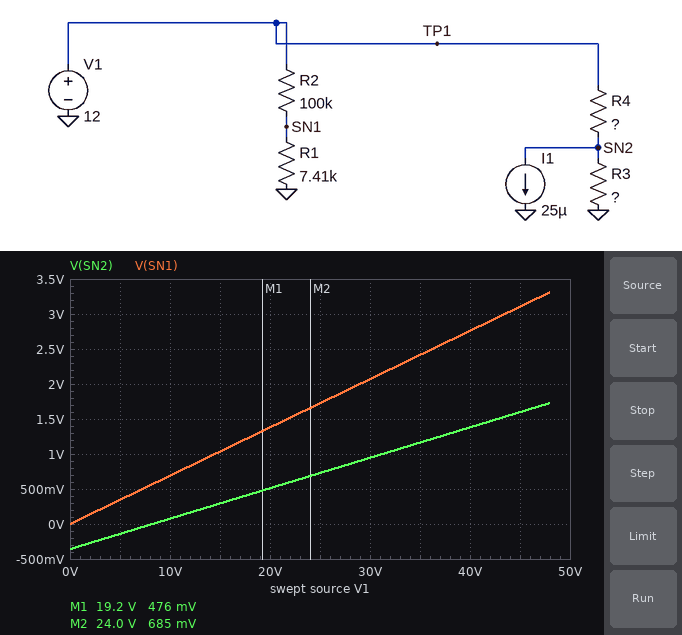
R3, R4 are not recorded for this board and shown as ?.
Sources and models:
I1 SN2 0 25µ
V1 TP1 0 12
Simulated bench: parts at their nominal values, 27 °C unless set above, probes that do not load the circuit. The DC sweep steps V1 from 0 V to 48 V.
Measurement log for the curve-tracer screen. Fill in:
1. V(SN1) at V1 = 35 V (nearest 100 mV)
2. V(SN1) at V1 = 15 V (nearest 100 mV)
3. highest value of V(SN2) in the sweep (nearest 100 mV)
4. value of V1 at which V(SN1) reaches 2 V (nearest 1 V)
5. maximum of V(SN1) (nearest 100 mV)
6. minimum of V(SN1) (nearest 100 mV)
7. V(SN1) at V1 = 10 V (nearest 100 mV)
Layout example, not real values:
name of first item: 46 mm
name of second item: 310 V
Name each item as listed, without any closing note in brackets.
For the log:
V(SN1) at V1 = 35 V: 2.4 V
V(SN1) at V1 = 15 V: 1.0 V
highest value of V(SN2) in the sweep: 1.7 V
value of V1 at which V(SN1) reaches 2 V: 29 V
maximum of V(SN1): 3.3 V
minimum of V(SN1): 0 V
V(SN1) at V1 = 10 V: 700 mV
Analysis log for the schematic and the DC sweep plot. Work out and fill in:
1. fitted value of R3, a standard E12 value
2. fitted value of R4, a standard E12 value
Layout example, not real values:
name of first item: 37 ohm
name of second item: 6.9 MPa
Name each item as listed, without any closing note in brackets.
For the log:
fitted value of R3, a standard E12 value: 15 kΩ
fitted value of R4, a standard E12 value: 330 kΩ
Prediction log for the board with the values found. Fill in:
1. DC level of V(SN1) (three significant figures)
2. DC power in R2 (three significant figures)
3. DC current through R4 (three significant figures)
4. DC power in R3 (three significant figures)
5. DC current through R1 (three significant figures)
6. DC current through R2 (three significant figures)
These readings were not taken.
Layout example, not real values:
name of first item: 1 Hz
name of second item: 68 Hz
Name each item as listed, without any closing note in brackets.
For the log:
DC level of V(SN1): 828 mV
DC power in R2: 1.25 mW
DC current through R4: 35.9 µA
DC power in R3: 1.77 µW
DC current through R1: 112 µA
DC current through R2: 112 µA
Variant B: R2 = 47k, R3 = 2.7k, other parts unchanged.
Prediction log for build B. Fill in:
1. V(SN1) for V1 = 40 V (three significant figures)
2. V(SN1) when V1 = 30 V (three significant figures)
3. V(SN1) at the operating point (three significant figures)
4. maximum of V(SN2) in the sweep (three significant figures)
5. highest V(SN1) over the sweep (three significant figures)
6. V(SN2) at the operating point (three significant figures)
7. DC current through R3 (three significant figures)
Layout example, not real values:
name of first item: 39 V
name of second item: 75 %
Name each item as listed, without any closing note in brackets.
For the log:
V(SN1) for V1 = 40 V: 5.45 V
V(SN1) when V1 = 30 V: 4.09 V
V(SN1) at the operating point: 1.63 V
maximum of V(SN2) in the sweep: 323 mV
highest V(SN1) over the sweep: 6.54 V
V(SN2) at the operating point: 30.4 mV
DC current through R3: 11.3 µA
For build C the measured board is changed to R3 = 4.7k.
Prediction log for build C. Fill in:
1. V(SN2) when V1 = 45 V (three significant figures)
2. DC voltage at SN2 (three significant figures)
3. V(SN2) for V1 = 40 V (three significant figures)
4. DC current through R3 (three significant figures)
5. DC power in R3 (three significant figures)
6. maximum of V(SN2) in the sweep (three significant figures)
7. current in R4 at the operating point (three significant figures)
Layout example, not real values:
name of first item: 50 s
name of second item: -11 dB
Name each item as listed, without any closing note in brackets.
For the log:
V(SN2) when V1 = 45 V: 516 mV
DC voltage at SN2: 52.7 mV
V(SN2) for V1 = 40 V: 446 mV
DC current through R3: 11.2 µA
DC power in R3: 590 nW
maximum of V(SN2) in the sweep: 558 mV
current in R4 at the operating point: 36.2 µA
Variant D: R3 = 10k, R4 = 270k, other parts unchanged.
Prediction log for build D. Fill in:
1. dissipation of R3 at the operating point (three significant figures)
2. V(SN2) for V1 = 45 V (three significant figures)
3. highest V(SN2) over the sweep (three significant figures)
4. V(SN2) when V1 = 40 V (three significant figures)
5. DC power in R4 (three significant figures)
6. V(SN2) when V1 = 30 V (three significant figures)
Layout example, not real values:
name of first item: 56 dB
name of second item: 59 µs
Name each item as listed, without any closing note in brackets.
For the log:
dissipation of R3 at the operating point: 3.52 µW
V(SN2) for V1 = 45 V: 1.37 V
highest V(SN2) over the sweep: 1.47 V
V(SN2) when V1 = 40 V: 1.19 V
DC power in R4: 517 µW
V(SN2) when V1 = 30 V: 830 mV
